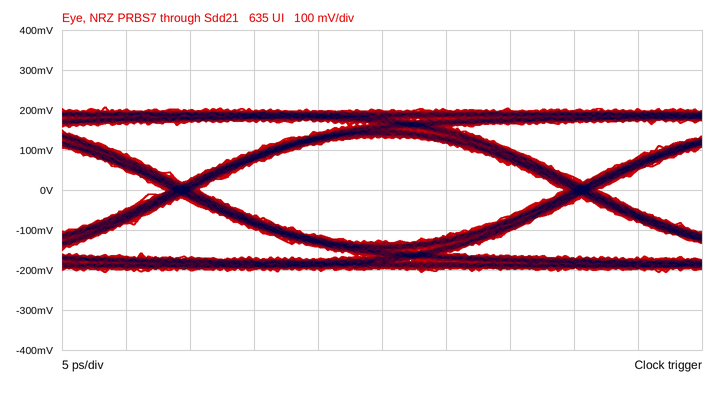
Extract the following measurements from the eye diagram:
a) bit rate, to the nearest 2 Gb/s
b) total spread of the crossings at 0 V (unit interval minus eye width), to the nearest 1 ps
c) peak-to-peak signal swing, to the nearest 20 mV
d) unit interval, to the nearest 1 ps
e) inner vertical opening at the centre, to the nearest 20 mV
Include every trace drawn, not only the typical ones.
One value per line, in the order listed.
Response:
32 Gb/s
3 ps
420 mV
31 ps
260 mV
